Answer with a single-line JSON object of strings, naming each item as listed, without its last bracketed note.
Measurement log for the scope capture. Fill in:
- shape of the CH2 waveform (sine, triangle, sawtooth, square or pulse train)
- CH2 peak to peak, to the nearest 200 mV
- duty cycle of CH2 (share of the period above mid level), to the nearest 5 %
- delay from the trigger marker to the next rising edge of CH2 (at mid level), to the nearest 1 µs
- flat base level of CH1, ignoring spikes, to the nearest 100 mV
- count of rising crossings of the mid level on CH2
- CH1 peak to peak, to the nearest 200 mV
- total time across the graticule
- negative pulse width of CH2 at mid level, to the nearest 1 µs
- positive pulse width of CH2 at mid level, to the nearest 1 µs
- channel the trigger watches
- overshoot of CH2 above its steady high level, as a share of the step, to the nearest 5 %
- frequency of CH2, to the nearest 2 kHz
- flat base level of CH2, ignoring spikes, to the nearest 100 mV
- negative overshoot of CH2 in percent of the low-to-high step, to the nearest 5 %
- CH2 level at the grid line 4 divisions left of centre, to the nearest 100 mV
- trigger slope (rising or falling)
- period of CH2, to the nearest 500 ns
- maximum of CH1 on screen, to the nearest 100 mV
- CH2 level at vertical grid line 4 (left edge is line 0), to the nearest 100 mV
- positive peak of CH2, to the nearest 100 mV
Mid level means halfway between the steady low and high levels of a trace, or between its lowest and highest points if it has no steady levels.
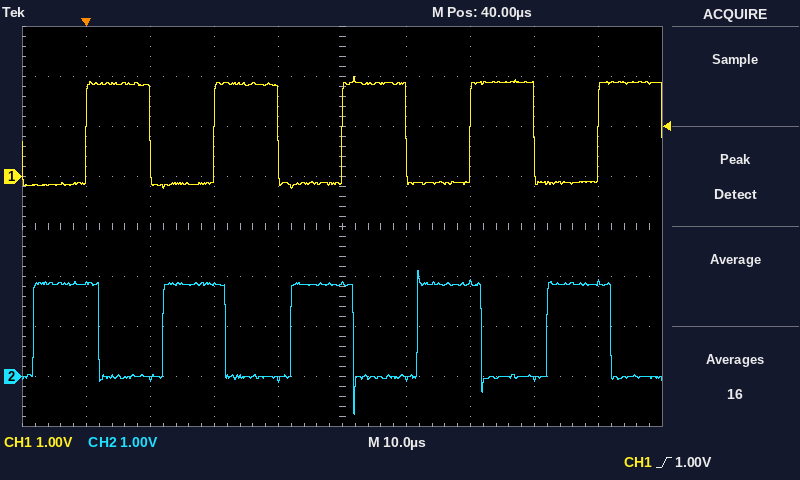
{"shape of the CH2 waveform": "square", "CH2 peak to peak, to the nearest 200 mV": "2.8 V", "duty cycle of CH2 (share of the period above mid level), to the nearest 5 %": "50 %", "delay from the trigger marker to the next rising edge of CH2 (at mid level), to the nearest 1 µs": "12 µs", "flat base level of CH1, ignoring spikes, to the nearest 100 mV": "-100 mV", "count of rising crossings of the mid level on CH2": "5", "CH1 peak to peak, to the nearest 200 mV": "2.2 V", "total time across the graticule": "100 µs", "negative pulse width of CH2 at mid level, to the nearest 1 µs": "10 µs", "positive pulse width of CH2 at mid level, to the nearest 1 µs": "10 µs", "channel the trigger watches": "CH1", "overshoot of CH2 above its steady high level, as a share of the step, to the nearest 5 %": "15 %", "frequency of CH2, to the nearest 2 kHz": "50 kHz", "flat base level of CH2, ignoring spikes, to the nearest 100 mV": "0.0 V", "negative overshoot of CH2 in percent of the low-to-high step, to the nearest 5 %": "40 %", "CH2 level at the grid line 4 divisions left of centre, to the nearest 100 mV": "1.9 V", "trigger slope": "rising", "period of CH2, to the nearest 500 ns": "20.0 µs", "maximum of CH1 on screen, to the nearest 100 mV": "2.0 V", "CH2 level at vertical grid line 4 (left edge is line 0), to the nearest 100 mV": "-100 mV", "positive peak of CH2, to the nearest 100 mV": "2.1 V"}
